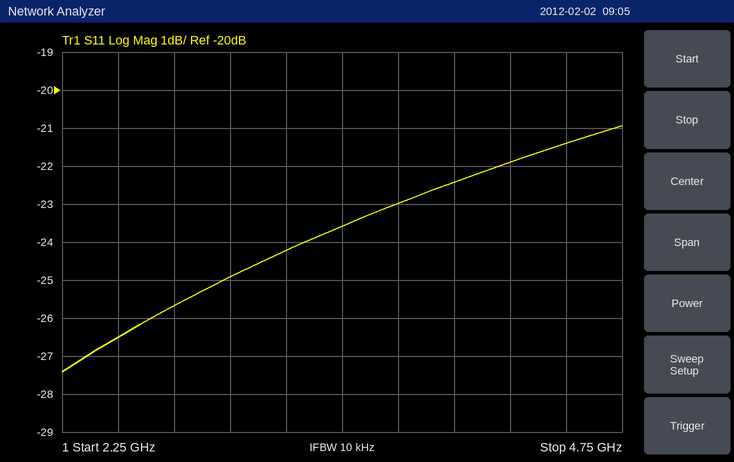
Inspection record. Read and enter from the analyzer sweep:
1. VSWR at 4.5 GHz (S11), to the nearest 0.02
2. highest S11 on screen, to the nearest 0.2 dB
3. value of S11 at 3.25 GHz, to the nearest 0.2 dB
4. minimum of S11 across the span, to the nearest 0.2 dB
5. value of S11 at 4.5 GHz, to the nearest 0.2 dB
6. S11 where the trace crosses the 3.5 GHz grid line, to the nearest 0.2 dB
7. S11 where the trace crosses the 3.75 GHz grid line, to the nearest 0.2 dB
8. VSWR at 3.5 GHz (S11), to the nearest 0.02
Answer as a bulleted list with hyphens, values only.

- 1.18
- -21.0 dB
- -24.2 dB
- -27.4 dB
- -21.4 dB
- -23.6 dB
- -23.0 dB
- 1.14
